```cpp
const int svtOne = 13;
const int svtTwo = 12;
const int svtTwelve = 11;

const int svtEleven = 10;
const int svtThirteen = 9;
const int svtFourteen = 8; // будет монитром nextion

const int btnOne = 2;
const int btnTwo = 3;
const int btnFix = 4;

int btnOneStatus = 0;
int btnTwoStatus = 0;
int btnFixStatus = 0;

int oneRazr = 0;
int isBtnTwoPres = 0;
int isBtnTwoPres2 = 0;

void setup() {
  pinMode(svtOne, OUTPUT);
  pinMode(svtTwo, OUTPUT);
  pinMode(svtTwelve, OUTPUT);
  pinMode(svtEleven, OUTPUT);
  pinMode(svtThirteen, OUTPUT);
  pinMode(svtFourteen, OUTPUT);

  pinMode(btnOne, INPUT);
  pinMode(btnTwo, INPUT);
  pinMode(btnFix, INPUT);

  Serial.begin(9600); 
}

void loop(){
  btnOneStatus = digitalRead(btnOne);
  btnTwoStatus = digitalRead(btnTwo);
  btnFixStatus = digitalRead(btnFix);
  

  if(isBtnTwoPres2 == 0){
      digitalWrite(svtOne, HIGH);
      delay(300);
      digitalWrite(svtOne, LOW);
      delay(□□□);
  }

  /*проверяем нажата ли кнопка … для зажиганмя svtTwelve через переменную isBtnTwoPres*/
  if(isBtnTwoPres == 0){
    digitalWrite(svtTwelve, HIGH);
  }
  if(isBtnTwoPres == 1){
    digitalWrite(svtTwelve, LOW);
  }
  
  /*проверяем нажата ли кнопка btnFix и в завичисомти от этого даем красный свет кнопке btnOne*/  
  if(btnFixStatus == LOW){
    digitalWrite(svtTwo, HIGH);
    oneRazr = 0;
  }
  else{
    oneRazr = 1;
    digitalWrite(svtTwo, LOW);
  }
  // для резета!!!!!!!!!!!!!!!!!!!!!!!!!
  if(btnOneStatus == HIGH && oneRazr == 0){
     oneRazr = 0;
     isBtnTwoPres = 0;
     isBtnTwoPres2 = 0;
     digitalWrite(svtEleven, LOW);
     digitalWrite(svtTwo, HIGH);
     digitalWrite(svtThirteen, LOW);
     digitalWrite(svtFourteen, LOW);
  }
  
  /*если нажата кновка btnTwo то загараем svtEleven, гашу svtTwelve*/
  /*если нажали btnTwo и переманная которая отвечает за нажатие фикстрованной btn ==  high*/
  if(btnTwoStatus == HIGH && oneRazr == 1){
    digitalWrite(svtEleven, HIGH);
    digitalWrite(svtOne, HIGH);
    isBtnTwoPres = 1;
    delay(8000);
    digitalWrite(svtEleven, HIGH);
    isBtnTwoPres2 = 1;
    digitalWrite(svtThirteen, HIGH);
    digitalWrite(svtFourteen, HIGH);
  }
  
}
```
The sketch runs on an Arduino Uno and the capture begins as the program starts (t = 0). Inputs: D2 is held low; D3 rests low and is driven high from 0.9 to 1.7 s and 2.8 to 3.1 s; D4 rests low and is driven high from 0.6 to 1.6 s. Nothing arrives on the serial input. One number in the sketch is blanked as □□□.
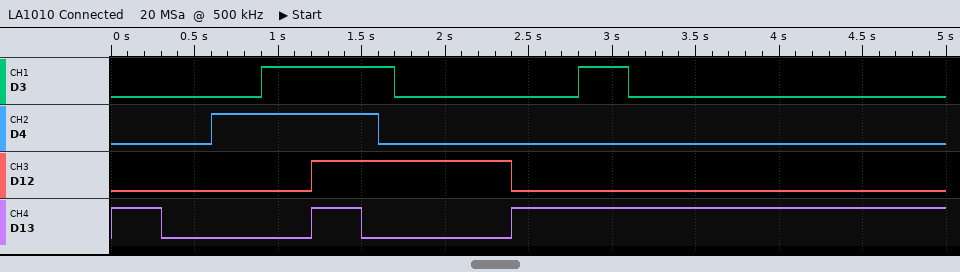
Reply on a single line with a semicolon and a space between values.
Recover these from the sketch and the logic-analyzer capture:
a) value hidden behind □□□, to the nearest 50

900
